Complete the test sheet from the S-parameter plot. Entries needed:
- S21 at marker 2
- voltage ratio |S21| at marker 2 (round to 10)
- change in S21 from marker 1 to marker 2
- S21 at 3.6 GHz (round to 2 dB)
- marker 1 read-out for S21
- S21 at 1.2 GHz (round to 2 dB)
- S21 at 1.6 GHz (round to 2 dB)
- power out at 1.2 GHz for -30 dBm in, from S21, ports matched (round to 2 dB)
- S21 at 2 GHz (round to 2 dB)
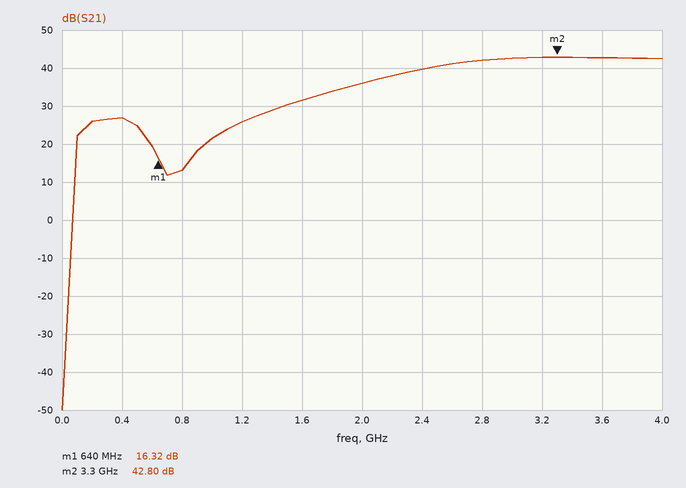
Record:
42.80 dB
140
26.48 dB
42 dB
16.32 dB
26 dB
32 dB
-4 dBm
36 dB
